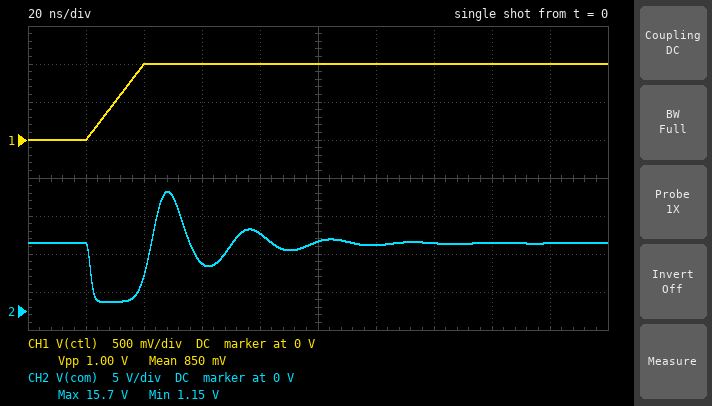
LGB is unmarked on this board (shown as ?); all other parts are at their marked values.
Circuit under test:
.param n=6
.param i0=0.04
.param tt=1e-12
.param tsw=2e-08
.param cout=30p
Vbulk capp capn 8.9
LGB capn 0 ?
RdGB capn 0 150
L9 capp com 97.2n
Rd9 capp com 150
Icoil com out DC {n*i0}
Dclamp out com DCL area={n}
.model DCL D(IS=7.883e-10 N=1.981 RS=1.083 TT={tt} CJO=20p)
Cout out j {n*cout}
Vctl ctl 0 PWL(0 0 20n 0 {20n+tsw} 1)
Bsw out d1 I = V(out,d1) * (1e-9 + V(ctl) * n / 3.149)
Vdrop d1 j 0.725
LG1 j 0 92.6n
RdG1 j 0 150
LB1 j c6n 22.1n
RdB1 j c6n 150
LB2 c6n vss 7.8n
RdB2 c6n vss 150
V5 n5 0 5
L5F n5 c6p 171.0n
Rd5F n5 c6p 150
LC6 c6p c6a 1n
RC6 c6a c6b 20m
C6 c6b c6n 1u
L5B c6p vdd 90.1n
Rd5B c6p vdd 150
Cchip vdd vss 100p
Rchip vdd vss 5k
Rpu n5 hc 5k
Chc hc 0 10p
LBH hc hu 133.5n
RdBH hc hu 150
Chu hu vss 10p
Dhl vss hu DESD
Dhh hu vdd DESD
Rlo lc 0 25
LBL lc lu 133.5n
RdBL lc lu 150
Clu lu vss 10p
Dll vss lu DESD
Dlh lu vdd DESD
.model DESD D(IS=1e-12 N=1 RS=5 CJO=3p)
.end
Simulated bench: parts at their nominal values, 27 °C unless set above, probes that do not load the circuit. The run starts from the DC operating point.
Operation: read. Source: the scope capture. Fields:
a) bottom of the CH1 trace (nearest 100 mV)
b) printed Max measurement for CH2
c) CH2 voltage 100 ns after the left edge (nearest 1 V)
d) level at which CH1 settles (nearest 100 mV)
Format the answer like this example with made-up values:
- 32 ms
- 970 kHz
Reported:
- 0 V
- 15.7 V
- 9 V
- 1.0 V
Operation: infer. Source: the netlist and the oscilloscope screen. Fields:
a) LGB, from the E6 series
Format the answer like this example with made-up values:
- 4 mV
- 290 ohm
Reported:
- 330 nH
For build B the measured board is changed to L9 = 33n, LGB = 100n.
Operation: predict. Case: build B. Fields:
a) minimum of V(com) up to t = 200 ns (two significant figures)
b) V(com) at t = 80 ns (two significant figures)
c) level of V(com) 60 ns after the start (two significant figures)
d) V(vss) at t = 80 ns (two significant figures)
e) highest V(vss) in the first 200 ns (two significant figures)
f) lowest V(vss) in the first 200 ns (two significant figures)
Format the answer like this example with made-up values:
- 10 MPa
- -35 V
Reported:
- 2.8 V
- 8.4 V
- 8.0 V
- 290 mV
- 2.2 V
- -2.5 V
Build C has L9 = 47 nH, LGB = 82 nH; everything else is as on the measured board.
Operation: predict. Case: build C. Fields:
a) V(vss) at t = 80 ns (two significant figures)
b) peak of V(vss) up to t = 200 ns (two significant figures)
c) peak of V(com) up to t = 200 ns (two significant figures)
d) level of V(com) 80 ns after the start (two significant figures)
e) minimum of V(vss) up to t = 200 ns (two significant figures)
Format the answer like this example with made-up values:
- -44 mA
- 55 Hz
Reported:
- 360 mV
- 2.3 V
- 16 V
- 8.3 V
- -2.6 V
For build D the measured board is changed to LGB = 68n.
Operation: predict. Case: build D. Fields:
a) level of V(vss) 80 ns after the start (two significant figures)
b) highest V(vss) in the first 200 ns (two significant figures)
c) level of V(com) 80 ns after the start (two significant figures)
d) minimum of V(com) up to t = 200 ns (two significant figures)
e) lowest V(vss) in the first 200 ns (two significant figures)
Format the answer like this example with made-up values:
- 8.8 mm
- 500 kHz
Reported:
- -220 mV
- 1.9 V
- 9.3 V
- 2.4 V
- -2.3 V
